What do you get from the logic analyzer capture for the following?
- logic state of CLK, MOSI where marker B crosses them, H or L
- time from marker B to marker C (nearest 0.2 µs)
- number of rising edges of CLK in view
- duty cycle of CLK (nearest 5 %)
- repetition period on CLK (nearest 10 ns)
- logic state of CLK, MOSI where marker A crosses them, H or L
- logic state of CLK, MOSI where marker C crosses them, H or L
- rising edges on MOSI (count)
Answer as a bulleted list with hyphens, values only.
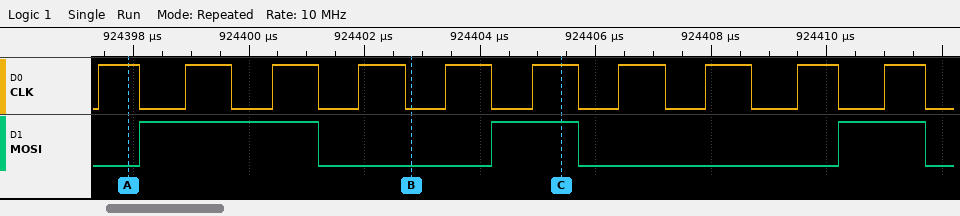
- CLK=L, MOSI=L
- 2.6 µs
- 10
- 50 %
- 1510 ns
- CLK=H, MOSI=L
- CLK=H, MOSI=H
- 3
